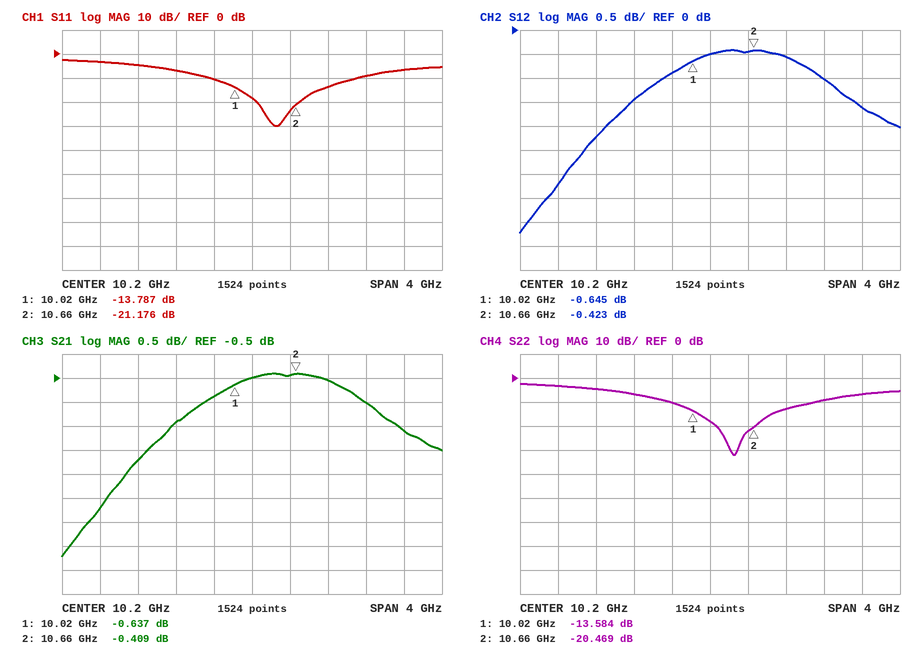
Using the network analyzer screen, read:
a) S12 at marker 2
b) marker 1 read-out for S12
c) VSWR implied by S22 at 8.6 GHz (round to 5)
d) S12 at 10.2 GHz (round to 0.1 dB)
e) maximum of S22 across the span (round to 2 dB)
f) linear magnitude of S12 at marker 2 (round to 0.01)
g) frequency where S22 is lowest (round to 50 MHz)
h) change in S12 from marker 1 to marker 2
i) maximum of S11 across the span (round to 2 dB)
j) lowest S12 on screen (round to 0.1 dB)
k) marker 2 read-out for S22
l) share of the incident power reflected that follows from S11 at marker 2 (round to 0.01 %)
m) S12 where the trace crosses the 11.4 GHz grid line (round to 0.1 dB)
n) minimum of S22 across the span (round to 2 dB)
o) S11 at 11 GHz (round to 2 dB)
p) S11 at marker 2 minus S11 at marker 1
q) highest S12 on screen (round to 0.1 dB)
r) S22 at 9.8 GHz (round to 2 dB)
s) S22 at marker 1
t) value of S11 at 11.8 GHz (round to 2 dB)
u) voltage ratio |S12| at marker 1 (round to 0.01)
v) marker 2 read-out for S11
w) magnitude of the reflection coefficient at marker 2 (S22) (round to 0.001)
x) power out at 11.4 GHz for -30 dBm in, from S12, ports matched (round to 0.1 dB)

-0.423 dB
-0.645 dB
5
-0.5 dB
-2 dB
0.95
10.45 GHz
0.222 dB
-2 dB
-4.2 dB
-20.469 dB
0.76 %
-1.0 dB
-32 dB
-14 dB
-7.389 dB
-0.4 dB
-10 dB
-13.584 dB
-6 dB
0.93
-21.176 dB
0.095
-31.0 dBm
